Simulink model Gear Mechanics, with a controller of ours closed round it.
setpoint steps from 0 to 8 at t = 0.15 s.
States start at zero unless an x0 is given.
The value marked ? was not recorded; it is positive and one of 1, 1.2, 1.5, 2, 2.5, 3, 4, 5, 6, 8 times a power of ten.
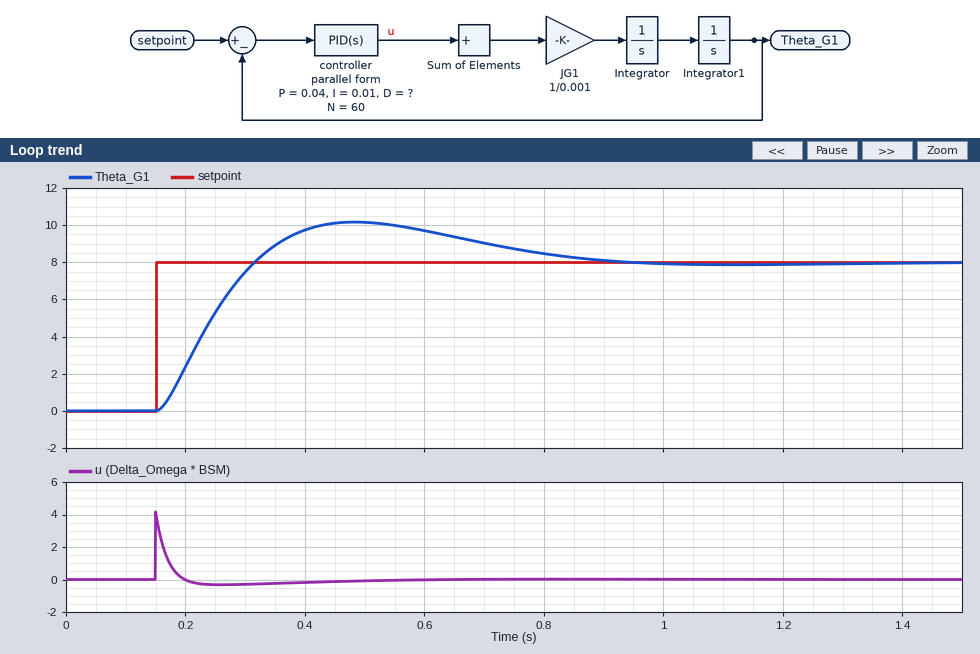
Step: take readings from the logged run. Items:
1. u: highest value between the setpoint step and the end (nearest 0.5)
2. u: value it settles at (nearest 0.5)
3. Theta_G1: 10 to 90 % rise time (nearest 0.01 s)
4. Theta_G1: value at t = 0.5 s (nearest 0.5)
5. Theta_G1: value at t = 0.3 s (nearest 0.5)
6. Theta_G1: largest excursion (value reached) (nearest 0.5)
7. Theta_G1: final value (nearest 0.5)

4.0
0.0
0.12 s
10.0
7.5
10.0
8.0
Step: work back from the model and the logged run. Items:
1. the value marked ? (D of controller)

0.008
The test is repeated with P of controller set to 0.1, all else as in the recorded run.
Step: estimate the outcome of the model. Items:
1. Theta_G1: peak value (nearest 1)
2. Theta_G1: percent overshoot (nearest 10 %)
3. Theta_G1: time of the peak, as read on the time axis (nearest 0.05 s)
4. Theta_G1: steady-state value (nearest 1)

11
40 %
0.40 s
8
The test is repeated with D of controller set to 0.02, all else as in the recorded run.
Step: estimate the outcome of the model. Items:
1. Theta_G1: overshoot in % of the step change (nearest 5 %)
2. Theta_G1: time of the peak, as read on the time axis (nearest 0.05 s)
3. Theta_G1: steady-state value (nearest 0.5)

10 %
0.30 s
8.0
